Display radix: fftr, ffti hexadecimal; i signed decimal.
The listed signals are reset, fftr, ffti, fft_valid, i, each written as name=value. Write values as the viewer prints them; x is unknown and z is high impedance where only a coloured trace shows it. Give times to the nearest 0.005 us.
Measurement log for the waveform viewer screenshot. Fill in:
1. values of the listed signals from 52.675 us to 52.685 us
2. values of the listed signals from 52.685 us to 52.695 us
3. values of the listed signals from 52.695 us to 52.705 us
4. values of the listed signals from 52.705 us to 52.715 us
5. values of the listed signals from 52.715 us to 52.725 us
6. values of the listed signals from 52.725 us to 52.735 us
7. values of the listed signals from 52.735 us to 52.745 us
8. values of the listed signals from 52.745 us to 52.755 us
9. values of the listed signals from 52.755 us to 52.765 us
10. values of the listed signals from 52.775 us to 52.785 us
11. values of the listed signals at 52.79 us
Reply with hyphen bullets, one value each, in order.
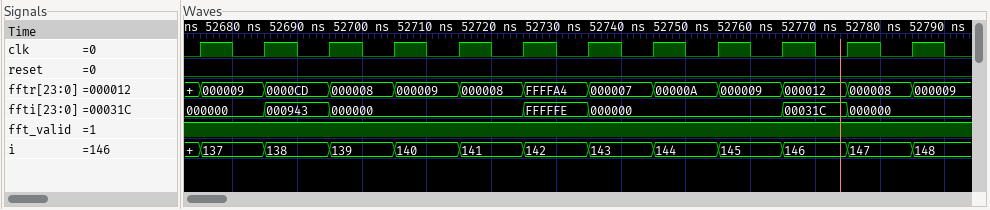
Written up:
- reset=0, fftr=000009, ffti=000000, fft_valid=1, i=137
- reset=0, fftr=0000CD, ffti=000943, fft_valid=1, i=138
- reset=0, fftr=000008, ffti=000000, fft_valid=1, i=139
- reset=0, fftr=000009, ffti=000000, fft_valid=1, i=140
- reset=0, fftr=000008, ffti=000000, fft_valid=1, i=141
- reset=0, fftr=FFFFA4, ffti=FFFFFE, fft_valid=1, i=142
- reset=0, fftr=000007, ffti=000000, fft_valid=1, i=143
- reset=0, fftr=00000A, ffti=000000, fft_valid=1, i=144
- reset=0, fftr=000009, ffti=000000, fft_valid=1, i=145
- reset=0, fftr=000008, ffti=000000, fft_valid=1, i=147
- reset=0, fftr=000009, ffti=000000, fft_valid=1, i=148
